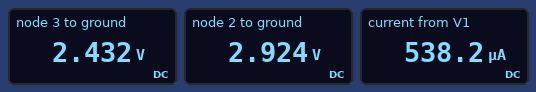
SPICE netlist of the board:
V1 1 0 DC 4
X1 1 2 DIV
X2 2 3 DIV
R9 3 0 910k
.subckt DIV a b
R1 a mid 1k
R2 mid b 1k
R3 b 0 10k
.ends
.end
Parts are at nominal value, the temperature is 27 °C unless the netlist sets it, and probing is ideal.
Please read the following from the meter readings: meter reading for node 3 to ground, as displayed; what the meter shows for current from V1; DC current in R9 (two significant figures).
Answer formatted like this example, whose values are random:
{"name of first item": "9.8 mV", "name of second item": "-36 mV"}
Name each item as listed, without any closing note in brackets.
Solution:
{"meter reading for node 3 to ground, as displayed": "2.432 V", "what the meter shows for current from V1": "538.2 µA", "DC current in R9": "2.7 µA"}
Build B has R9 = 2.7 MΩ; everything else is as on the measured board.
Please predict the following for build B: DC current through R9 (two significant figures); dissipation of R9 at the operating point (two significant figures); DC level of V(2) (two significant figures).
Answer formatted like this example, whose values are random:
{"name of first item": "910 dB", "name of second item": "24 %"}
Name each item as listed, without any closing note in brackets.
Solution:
{"DC current through R9": "900 nA", "dissipation of R9 at the operating point": "2.2 µW", "DC level of V(2)": "2.9 V"}
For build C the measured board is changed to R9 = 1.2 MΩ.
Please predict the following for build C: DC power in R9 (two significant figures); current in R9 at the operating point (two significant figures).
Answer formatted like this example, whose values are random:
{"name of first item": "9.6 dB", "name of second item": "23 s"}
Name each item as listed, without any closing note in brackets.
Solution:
{"DC power in R9": "4.9 µW", "current in R9 at the operating point": "2.0 µA"}
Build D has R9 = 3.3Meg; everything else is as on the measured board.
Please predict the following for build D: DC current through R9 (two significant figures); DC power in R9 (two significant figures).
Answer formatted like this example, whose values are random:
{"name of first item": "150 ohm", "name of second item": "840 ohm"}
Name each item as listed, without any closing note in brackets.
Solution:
{"DC current through R9": "740 nA", "DC power in R9": "1.8 µW"}
